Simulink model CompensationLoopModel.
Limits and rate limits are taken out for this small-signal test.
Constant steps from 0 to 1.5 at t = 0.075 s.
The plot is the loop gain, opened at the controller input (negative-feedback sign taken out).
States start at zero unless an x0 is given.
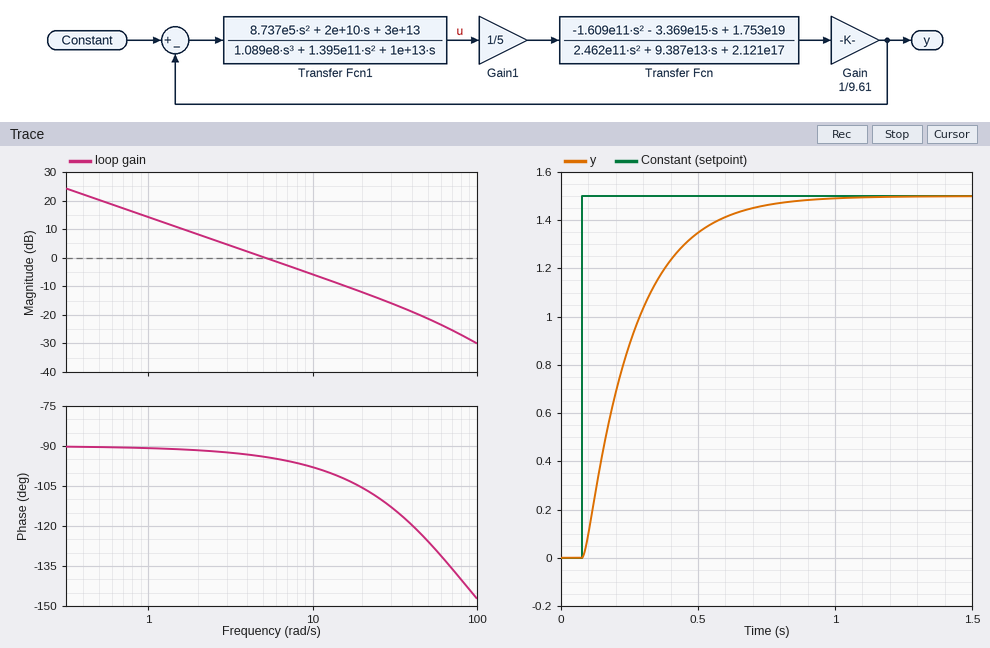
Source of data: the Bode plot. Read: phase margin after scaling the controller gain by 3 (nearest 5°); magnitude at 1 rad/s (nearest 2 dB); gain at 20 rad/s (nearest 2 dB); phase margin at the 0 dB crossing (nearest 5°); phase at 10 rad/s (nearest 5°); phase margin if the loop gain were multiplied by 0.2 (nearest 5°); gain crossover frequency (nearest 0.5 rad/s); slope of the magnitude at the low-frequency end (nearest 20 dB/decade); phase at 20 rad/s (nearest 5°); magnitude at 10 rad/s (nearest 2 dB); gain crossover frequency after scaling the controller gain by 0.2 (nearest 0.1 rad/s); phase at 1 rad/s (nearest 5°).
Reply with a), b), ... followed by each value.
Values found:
a) 80°
b) 14 dB
c) -12 dB
d) 85°
e) -100°
f) 90°
g) 5.0 rad/s
h) -20 dB/decade
i) -105°
j) -6 dB
k) 1.0 rad/s
l) -90°
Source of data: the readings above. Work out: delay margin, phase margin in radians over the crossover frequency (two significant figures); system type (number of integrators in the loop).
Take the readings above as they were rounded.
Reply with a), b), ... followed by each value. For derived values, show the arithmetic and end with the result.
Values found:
a) 85 × π / 180 / 5 = 0.30 s
b) 1
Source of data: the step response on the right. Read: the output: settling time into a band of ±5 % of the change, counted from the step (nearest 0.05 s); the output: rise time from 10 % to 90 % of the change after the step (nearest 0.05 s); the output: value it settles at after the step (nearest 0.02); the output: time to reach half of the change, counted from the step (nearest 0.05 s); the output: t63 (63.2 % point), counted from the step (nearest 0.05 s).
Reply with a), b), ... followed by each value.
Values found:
a) 0.55 s
b) 0.40 s
c) 1.50
d) 0.15 s
e) 0.20 s
